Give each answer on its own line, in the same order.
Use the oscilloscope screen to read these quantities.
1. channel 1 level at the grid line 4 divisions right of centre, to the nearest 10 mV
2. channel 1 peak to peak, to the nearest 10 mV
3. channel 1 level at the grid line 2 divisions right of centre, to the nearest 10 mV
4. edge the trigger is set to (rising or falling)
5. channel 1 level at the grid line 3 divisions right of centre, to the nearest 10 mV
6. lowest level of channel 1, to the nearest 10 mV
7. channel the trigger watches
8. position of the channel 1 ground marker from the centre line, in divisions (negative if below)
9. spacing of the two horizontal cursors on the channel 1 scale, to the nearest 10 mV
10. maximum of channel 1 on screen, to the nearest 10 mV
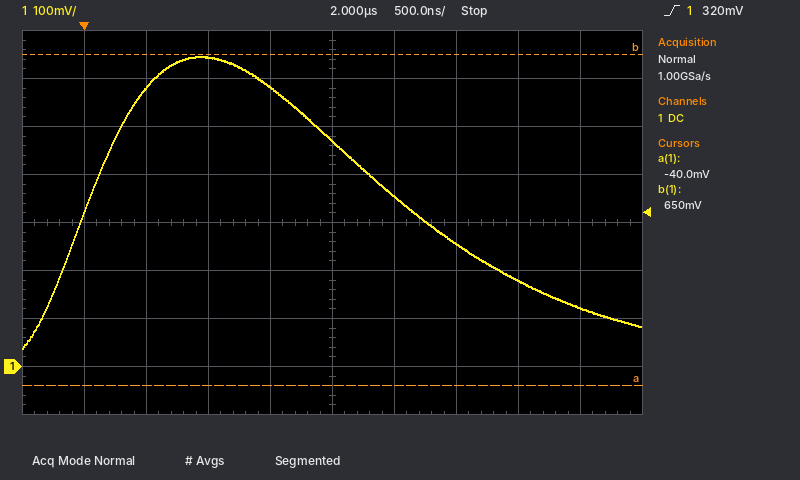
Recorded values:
120 mV
610 mV
260 mV
rising
180 mV
40 mV
channel 1
-3.0 div
690 mV
650 mV
